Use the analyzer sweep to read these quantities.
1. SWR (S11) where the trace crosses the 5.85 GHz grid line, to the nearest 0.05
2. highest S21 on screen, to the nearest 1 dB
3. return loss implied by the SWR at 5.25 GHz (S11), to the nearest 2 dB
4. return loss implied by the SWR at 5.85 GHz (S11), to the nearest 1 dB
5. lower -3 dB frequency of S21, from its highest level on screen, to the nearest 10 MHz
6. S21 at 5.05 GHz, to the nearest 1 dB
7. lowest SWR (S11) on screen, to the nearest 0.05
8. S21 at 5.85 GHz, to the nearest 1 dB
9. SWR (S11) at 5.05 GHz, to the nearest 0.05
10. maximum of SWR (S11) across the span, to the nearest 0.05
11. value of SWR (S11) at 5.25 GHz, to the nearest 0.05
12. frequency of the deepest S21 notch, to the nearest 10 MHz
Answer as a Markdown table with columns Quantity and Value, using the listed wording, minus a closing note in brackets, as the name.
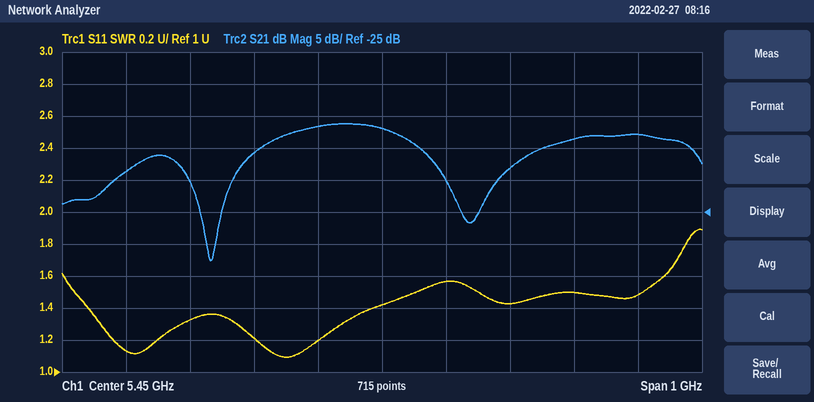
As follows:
| Quantity | Value |
|---|---|
| SWR (S11) where the trace crosses the 5.85 GHz grid line, to the nearest 0.05 | 1.50 |
| highest S21 on screen, to the nearest 1 dB | -11 dB |
| return loss implied by the SWR at 5.25 GHz (S11), to the nearest 2 dB | 20 dB |
| return loss implied by the SWR at 5.85 GHz (S11), to the nearest 1 dB | 14 dB |
| lower -3 dB frequency of S21, from its highest level on screen, to the nearest 10 MHz | 5.27 GHz |
| S21 at 5.05 GHz, to the nearest 1 dB | -19 dB |
| lowest SWR (S11) on screen, to the nearest 0.05 | 1.10 |
| S21 at 5.85 GHz, to the nearest 1 dB | -13 dB |
| SWR (S11) at 5.05 GHz, to the nearest 0.05 | 1.15 |
| maximum of SWR (S11) across the span, to the nearest 0.05 | 1.90 |
| value of SWR (S11) at 5.25 GHz, to the nearest 0.05 | 1.20 |
| frequency of the deepest S21 notch, to the nearest 10 MHz | 5.18 GHz |
